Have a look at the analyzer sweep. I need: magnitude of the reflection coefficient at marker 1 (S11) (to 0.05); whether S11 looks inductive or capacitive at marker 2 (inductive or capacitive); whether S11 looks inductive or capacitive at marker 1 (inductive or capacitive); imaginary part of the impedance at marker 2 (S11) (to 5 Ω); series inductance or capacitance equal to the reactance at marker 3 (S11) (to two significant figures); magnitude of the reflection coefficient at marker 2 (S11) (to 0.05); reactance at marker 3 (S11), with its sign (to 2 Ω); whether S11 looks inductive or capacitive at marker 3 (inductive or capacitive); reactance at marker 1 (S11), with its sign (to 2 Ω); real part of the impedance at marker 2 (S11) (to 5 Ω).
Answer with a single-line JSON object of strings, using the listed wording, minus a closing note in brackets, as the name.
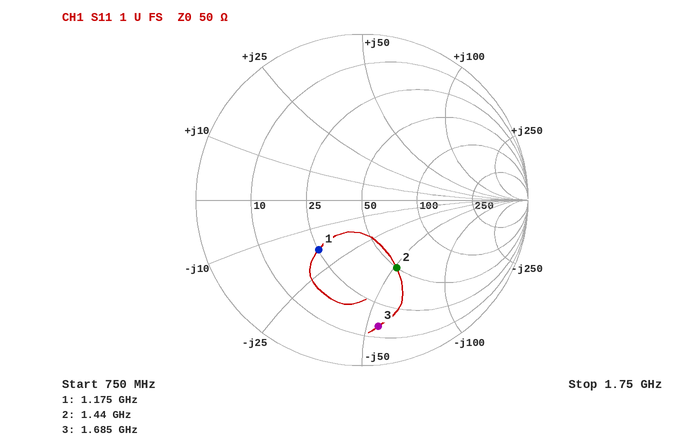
{"magnitude of the reflection coefficient at marker 1 (S11)": "0.40", "whether S11 looks inductive or capacitive at marker 2": "capacitive", "whether S11 looks inductive or capacitive at marker 1": "capacitive", "imaginary part of the impedance at marker 2 (S11)": "-50 Ω", "series inductance or capacitance equal to the reactance at marker 3 (S11)": "1.7 pF", "magnitude of the reflection coefficient at marker 2 (S11)": "0.45", "reactance at marker 3 (S11), with its sign": "-54 Ω", "whether S11 looks inductive or capacitive at marker 3": "capacitive", "reactance at marker 1 (S11), with its sign": "-18 Ω", "real part of the impedance at marker 2 (S11)": "50 Ω"}
